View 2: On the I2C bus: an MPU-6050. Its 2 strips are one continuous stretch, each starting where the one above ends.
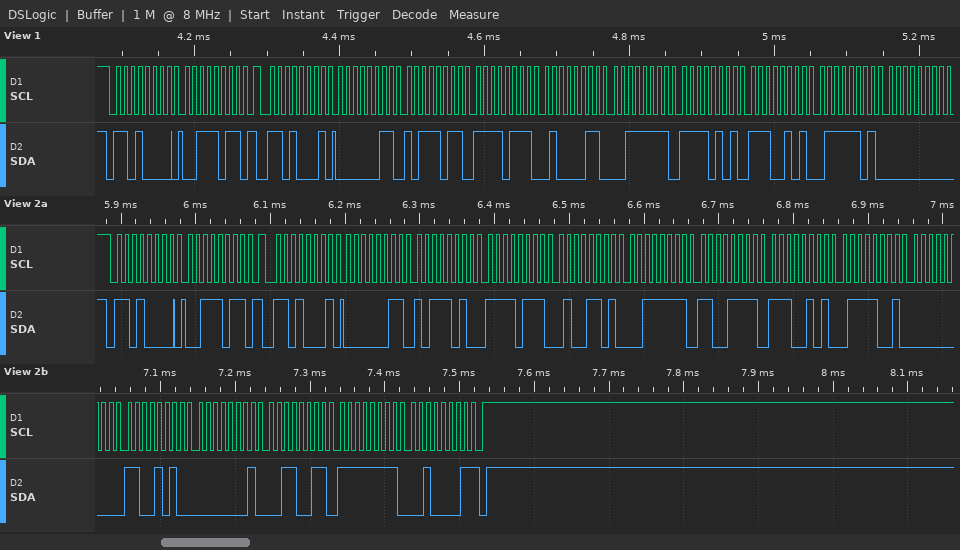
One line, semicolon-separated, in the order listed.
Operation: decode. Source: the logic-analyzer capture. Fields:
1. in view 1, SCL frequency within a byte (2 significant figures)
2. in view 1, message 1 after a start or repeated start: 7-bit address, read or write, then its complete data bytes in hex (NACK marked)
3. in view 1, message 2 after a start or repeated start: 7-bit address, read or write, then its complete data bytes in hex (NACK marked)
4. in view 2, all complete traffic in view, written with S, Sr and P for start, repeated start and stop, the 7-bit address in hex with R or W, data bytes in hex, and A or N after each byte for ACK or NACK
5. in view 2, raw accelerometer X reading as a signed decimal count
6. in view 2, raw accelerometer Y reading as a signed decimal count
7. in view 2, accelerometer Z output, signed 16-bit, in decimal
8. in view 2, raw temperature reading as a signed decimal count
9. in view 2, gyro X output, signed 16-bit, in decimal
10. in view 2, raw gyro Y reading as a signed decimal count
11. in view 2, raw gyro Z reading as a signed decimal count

100 kHz; 0x68 write: 3B; 0x68 read: 03 BB F7 43 3F F5 E5 7D 00; S 68W A 3B A Sr 68R A 03 A BA A F7 A 4D A 3F A CF A E5 A 79 A 00 A CA A 01 A 33 A FF A 21 N P; 954; -2227; 16335; -6791; 202; 307; -223
